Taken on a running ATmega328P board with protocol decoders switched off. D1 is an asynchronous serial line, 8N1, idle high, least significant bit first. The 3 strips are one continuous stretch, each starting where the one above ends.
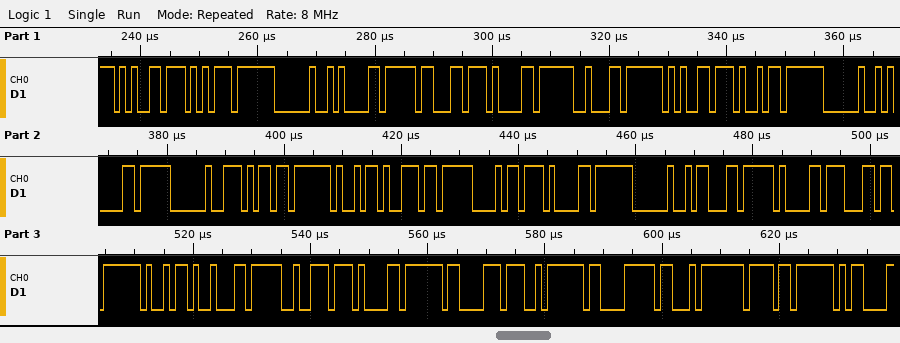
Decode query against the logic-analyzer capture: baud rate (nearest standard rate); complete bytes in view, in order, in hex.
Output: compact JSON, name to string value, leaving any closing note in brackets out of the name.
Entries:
{"baud rate": "1000000 baud", "complete bytes in view, in order, in hex": "0x65 0x75 0x20 0x61 0x63 0x61 0x62 0x65 0x69 0x20 0x61 0x20 0x6D 0x69 0x6E 0x68 0x61 0x20 0x63 0x61 0x6C 0x69 0x62 0x72 0x61 0xC3 0xA7 0xC3 0xA3 0x6F 0x0D"}
